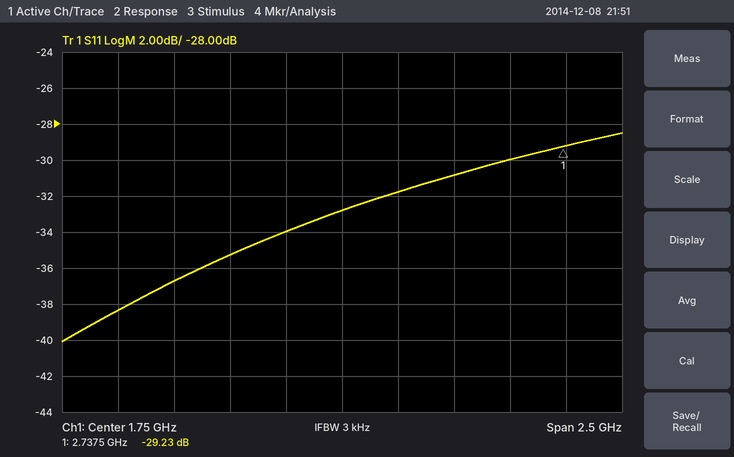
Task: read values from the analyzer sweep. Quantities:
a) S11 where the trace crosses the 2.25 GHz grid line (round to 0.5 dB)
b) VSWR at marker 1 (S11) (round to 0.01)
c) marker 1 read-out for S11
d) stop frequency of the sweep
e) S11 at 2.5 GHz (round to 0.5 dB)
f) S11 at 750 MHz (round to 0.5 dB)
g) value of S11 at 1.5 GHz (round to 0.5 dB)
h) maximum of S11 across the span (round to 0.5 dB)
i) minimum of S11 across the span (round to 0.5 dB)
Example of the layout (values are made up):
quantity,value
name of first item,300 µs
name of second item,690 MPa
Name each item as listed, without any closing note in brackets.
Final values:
quantity,value
S11 where the trace crosses the 2.25 GHz grid line,-31.0 dB
VSWR at marker 1 (S11),1.07
marker 1 read-out for S11,-29.23 dB
stop frequency of the sweep,3 GHz
S11 at 2.5 GHz,-30.0 dB
S11 at 750 MHz,-38.5 dB
value of S11 at 1.5 GHz,-34.0 dB
maximum of S11 across the span,-28.5 dB
minimum of S11 across the span,-40.0 dB
